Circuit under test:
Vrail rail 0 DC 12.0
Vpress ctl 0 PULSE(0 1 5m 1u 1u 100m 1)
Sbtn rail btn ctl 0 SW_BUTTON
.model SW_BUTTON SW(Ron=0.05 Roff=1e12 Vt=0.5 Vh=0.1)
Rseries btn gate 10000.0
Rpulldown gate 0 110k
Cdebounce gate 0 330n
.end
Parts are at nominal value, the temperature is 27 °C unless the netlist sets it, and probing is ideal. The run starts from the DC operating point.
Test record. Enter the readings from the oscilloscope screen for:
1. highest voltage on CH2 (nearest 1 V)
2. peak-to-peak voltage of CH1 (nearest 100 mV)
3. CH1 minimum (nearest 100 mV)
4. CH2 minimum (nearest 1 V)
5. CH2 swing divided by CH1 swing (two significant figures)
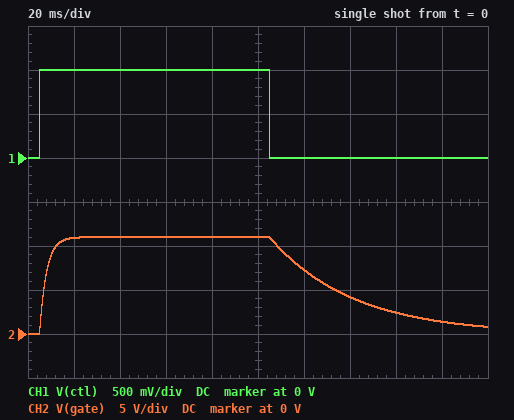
11 V
1.0 V
0 V
0 V
11
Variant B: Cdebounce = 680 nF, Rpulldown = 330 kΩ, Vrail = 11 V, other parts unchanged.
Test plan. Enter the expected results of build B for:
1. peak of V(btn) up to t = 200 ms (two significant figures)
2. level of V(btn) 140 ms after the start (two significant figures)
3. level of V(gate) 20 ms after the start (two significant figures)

11 V
9.1 V
9.6 V
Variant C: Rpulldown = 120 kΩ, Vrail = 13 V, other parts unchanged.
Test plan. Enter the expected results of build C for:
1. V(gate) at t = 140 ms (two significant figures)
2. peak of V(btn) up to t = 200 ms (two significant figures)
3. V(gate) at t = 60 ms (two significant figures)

5.0 V
13 V
12 V
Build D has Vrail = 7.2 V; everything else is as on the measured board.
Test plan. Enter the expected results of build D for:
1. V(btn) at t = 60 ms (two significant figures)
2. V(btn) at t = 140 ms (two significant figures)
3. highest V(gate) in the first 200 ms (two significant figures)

7.2 V
2.5 V
6.6 V
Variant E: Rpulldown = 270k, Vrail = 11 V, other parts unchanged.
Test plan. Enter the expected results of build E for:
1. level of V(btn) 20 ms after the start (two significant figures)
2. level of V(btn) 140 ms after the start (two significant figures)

11 V
7.2 V
